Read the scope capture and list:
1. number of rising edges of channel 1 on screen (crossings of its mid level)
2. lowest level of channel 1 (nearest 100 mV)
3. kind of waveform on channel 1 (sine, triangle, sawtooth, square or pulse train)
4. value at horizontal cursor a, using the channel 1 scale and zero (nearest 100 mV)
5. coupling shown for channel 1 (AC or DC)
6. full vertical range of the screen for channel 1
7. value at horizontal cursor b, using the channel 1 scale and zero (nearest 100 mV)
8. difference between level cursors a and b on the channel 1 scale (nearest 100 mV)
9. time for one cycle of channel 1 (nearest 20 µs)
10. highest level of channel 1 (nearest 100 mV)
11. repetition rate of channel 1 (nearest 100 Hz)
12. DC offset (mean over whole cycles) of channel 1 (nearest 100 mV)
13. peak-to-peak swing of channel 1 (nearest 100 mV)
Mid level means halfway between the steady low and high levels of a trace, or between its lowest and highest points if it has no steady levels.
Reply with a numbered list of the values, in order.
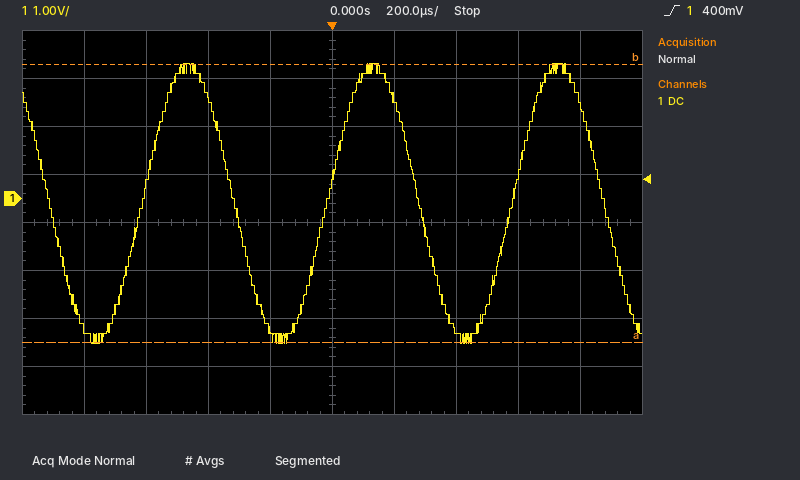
1. 3
2. -3.0 V
3. sine
4. -3.0 V
5. DC
6. 8 V
7. 2.8 V
8. 5.8 V
9. 600 µs
10. 2.8 V
11. 1.7 kHz
12. -100 mV
13. 5.8 V
